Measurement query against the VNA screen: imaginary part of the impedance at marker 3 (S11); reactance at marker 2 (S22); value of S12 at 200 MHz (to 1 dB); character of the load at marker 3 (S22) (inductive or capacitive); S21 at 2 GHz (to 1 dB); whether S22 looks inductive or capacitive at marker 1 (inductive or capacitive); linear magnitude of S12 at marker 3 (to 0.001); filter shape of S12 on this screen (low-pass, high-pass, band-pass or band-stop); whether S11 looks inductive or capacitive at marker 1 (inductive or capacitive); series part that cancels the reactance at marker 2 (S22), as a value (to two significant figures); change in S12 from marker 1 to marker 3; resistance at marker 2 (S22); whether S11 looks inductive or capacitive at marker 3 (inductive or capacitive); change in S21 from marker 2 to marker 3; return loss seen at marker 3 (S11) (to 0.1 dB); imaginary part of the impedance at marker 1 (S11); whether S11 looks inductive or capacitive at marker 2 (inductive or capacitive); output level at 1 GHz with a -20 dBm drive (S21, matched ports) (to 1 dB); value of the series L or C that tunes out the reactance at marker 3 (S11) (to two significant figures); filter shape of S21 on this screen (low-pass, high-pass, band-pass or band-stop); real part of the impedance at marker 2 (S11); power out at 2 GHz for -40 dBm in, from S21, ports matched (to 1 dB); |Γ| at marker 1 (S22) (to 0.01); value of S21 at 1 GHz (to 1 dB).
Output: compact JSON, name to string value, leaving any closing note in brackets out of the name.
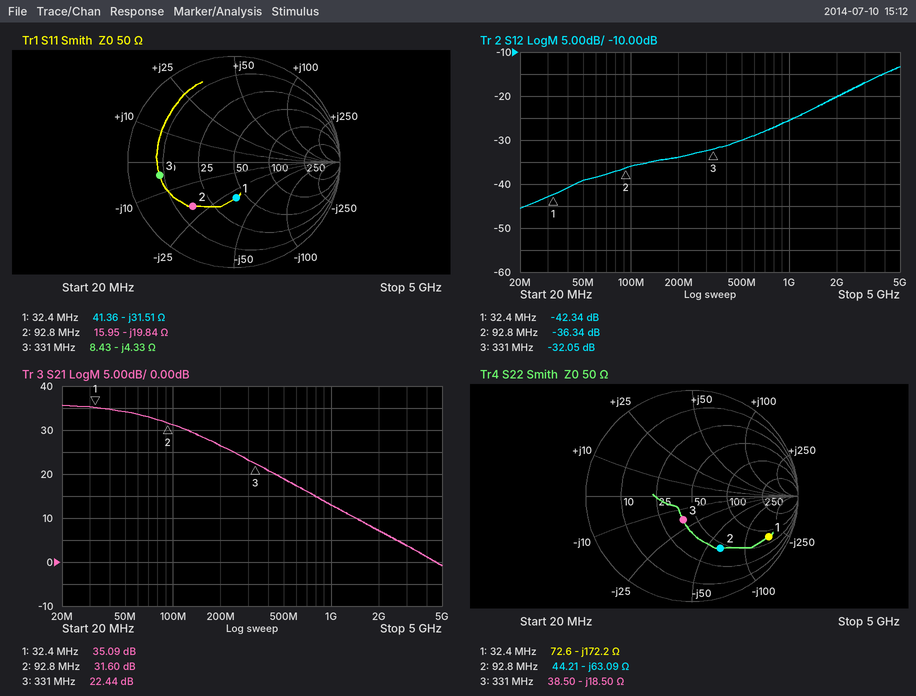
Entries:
{"imaginary part of the impedance at marker 3": "-4.33 Ω", "reactance at marker 2": "-63.09 Ω", "value of S12 at 200 MHz": "-34 dB", "character of the load at marker 3 (S22)": "capacitive", "S21 at 2 GHz": "7 dB", "whether S22 looks inductive or capacitive at marker 1": "capacitive", "linear magnitude of S12 at marker 3": "0.025", "filter shape of S12 on this screen": "high-pass", "whether S11 looks inductive or capacitive at marker 1": "capacitive", "series part that cancels the reactance at marker 2 (S22), as a value": "110 nH", "change in S12 from marker 1 to marker 3": "10.29 dB", "resistance at marker 2": "44.21 Ω", "whether S11 looks inductive or capacitive at marker 3": "capacitive", "change in S21 from marker 2 to marker 3": "-9.16 dB", "return loss seen at marker 3 (S11)": "2.9 dB", "imaginary part of the impedance at marker 1": "-31.51 Ω", "whether S11 looks inductive or capacitive at marker 2": "capacitive", "output level at 1 GHz with a -20 dBm drive (S21, matched ports)": "-7 dBm", "value of the series L or C that tunes out the reactance at marker 3 (S11)": "2.1 nH", "filter shape of S21 on this screen": "low-pass", "real part of the impedance at marker 2": "15.95 Ω", "power out at 2 GHz for -40 dBm in, from S21, ports matched": "-33 dBm", "|Γ| at marker 1 (S22)": "0.82", "value of S21 at 1 GHz": "13 dB"}
